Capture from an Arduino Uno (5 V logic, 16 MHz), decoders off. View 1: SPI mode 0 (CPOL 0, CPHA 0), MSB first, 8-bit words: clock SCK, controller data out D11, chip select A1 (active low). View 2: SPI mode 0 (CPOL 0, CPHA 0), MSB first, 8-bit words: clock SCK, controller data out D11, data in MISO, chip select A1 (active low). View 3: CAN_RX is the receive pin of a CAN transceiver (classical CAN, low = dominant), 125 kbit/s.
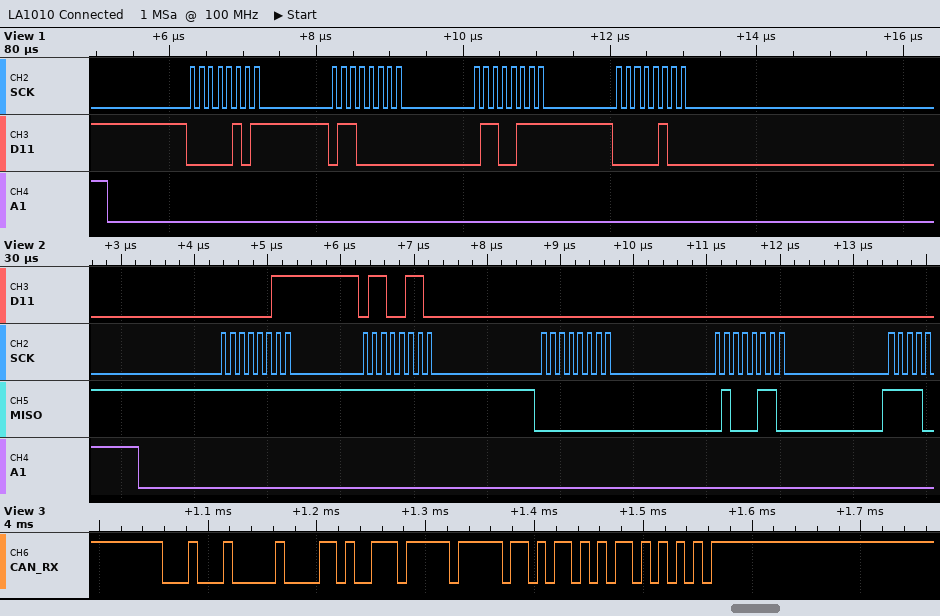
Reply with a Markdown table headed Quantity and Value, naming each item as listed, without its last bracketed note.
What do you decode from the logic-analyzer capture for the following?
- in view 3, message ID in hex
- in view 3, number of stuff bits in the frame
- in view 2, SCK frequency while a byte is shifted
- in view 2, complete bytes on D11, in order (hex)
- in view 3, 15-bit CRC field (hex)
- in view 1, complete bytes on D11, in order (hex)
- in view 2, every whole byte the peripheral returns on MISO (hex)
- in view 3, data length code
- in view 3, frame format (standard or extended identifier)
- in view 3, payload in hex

| Quantity | Value |
|---|---|
| in view 3, message ID in hex | 0x110 |
| in view 3, number of stuff bits in the frame | 3 |
| in view 2, SCK frequency while a byte is shifted | 8 MHz |
| in view 2, complete bytes on D11, in order | 03 66 00 00 |
| in view 3, 15-bit CRC field | 0x55AA |
| in view 1, complete bytes on D11, in order | 0x05 0x60 0x67 0x04 |
| in view 2, every whole byte the peripheral returns on MISO | FF FF 00 46 |
| in view 3, data length code | 3 |
| in view 3, frame format | standard |
| in view 3, payload in hex | 4E FF F5 |
